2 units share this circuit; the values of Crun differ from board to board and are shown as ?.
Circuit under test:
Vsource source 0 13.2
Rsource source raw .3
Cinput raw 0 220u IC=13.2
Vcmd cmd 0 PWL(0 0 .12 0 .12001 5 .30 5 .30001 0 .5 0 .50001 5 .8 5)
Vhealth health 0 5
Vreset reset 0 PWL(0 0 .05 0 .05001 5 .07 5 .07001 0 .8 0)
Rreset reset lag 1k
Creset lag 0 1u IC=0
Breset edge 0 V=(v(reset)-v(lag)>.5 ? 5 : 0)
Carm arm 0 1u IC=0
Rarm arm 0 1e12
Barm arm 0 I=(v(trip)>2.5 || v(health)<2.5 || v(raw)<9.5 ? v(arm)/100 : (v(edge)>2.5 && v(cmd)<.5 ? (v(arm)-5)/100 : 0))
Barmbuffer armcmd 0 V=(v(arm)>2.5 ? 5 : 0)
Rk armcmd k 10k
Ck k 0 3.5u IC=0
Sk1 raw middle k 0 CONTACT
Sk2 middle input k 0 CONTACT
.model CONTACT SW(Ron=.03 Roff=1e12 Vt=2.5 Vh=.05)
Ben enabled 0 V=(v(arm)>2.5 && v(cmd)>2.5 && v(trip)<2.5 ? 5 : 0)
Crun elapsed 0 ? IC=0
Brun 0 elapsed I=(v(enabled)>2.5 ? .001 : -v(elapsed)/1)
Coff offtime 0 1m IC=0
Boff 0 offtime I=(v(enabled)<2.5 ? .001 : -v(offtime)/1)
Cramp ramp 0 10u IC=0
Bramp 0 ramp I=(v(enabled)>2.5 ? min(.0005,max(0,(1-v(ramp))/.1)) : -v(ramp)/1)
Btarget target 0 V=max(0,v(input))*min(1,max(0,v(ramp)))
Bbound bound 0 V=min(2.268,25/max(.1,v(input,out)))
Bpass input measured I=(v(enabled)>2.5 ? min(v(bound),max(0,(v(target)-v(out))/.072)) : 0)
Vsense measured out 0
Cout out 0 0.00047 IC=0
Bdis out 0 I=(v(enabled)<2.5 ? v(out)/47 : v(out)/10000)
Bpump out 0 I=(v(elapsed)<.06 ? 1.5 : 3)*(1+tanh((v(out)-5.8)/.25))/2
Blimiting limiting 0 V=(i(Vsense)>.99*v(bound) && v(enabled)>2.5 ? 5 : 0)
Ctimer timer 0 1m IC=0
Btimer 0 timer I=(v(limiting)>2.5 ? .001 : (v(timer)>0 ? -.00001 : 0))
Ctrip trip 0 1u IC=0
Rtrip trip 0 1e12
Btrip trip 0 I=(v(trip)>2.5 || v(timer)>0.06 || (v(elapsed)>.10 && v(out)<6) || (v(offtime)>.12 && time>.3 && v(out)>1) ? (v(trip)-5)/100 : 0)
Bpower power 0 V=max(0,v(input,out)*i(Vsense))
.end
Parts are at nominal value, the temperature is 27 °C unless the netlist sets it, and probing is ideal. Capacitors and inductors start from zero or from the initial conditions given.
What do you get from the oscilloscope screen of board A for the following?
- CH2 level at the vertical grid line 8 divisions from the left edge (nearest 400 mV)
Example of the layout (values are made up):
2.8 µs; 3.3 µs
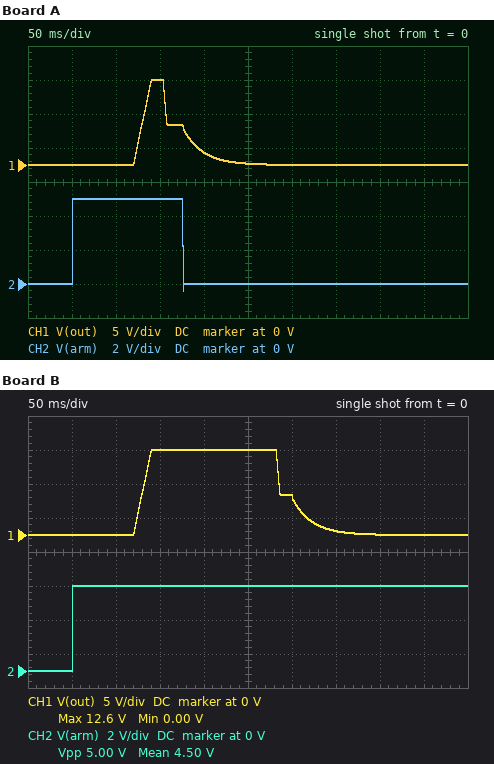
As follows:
0 V
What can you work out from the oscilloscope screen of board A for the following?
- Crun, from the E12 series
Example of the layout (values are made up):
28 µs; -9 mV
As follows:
560 µF
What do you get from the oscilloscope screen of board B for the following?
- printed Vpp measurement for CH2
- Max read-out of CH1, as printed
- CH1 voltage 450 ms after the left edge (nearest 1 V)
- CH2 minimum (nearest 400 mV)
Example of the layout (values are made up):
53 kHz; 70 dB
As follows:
5.00 V; 12.6 V; 0 V; 0 V
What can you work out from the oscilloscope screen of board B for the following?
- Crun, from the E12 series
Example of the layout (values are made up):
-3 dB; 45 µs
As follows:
2.7 mF
